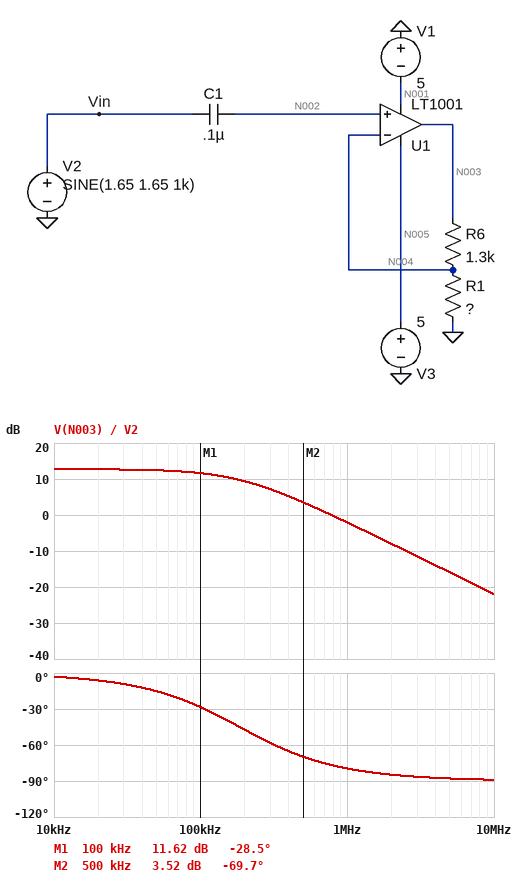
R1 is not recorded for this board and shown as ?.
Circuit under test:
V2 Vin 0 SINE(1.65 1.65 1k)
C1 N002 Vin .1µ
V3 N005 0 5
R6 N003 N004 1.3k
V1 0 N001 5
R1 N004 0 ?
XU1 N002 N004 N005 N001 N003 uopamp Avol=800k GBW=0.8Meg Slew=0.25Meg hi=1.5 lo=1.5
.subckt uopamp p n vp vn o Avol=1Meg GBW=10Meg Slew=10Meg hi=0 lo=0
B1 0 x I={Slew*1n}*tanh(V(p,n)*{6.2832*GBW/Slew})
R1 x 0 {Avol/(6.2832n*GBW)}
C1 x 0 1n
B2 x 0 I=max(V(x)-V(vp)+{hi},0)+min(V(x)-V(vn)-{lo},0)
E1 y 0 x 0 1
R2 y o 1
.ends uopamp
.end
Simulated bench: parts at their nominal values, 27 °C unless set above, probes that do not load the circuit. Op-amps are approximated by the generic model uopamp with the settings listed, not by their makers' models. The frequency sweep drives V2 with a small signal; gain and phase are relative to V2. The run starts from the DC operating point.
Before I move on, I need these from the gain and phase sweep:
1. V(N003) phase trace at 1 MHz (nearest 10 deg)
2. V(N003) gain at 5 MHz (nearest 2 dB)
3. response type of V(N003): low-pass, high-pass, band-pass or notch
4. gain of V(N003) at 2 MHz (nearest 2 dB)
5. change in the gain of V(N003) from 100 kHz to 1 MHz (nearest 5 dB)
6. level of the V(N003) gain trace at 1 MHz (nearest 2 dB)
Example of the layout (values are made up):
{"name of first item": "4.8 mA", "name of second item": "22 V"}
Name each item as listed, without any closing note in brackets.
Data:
{"V(N003) phase trace at 1 MHz": "-80 deg", "V(N003) gain at 5 MHz": "-16 dB", "response type of V(N003): low-pass, high-pass, band-pass or notch": "low-pass", "gain of V(N003) at 2 MHz": "-8 dB", "change in the gain of V(N003) from 100 kHz to 1 MHz": "-15 dB", "level of the V(N003) gain trace at 1 MHz": "-2 dB"}
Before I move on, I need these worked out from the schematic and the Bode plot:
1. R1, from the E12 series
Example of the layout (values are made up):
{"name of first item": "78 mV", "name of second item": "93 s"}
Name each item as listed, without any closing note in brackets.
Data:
{"R1, from the E12 series": "390 Ω"}
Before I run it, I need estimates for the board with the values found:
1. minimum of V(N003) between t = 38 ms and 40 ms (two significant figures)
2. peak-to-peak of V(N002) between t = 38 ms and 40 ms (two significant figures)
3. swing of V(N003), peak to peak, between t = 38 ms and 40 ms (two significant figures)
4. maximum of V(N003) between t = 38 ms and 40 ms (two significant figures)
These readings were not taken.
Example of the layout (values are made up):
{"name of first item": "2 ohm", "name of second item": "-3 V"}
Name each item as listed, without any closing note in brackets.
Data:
{"minimum of V(N003) between t = 38 ms and 40 ms": "-3.5 V", "peak-to-peak of V(N002) between t = 38 ms and 40 ms": "3.3 V", "swing of V(N003), peak to peak, between t = 38 ms and 40 ms": "7.0 V", "maximum of V(N003) between t = 38 ms and 40 ms": "3.5 V"}
